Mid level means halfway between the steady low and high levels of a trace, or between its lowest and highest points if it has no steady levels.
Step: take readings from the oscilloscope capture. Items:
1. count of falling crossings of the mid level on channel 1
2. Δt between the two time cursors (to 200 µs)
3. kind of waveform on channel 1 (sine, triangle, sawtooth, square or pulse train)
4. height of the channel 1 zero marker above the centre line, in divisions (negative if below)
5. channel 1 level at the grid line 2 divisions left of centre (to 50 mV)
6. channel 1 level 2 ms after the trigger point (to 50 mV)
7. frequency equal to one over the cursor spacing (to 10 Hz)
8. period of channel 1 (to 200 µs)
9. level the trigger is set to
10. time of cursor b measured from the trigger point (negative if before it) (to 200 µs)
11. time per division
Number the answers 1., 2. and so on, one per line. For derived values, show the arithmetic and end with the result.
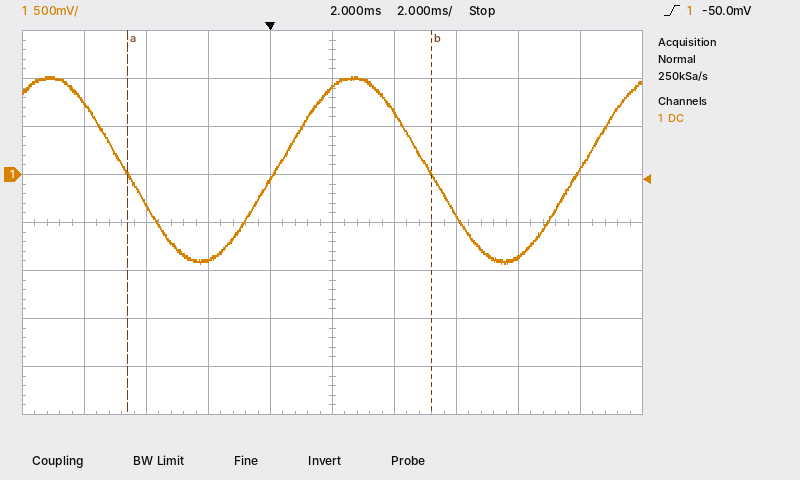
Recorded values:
1. 2
2. 9.8 ms
3. sine
4. +1.0 div
5. -900 mV
6. 900 mV
7. 1 / 9.8 ms ≈ 100 Hz
8. 9.8 ms
9. -50.0 mV
10. +5.2 ms
11. 2 ms
